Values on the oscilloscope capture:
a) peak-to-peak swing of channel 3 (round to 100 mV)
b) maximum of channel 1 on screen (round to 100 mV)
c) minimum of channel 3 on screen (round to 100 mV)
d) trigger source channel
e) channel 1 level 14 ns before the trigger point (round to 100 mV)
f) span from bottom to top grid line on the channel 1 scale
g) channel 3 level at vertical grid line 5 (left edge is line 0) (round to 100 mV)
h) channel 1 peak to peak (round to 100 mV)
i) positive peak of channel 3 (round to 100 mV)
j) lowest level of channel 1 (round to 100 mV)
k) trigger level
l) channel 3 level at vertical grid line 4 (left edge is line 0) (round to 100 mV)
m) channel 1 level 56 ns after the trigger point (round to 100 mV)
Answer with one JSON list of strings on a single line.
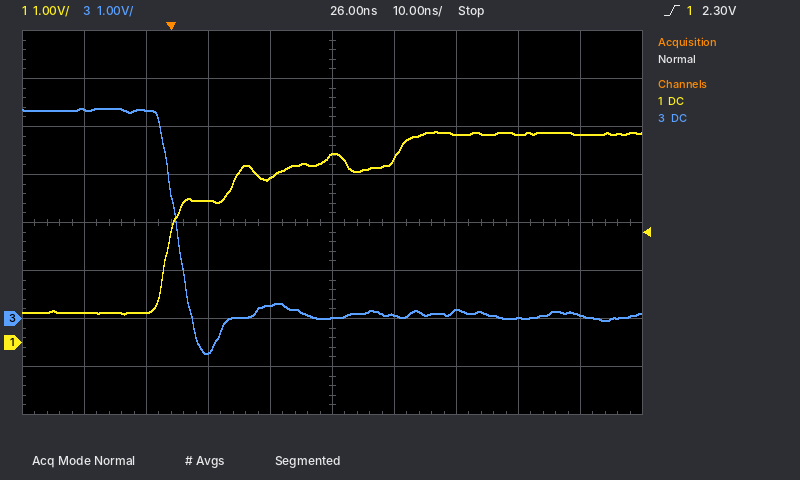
["5.1 V", "4.4 V", "-700 mV", "channel 1", "600 mV", "8 V", "0.0 V", "3.8 V", "4.4 V", "600 mV", "2.30 V", "300 mV", "4.3 V"]
